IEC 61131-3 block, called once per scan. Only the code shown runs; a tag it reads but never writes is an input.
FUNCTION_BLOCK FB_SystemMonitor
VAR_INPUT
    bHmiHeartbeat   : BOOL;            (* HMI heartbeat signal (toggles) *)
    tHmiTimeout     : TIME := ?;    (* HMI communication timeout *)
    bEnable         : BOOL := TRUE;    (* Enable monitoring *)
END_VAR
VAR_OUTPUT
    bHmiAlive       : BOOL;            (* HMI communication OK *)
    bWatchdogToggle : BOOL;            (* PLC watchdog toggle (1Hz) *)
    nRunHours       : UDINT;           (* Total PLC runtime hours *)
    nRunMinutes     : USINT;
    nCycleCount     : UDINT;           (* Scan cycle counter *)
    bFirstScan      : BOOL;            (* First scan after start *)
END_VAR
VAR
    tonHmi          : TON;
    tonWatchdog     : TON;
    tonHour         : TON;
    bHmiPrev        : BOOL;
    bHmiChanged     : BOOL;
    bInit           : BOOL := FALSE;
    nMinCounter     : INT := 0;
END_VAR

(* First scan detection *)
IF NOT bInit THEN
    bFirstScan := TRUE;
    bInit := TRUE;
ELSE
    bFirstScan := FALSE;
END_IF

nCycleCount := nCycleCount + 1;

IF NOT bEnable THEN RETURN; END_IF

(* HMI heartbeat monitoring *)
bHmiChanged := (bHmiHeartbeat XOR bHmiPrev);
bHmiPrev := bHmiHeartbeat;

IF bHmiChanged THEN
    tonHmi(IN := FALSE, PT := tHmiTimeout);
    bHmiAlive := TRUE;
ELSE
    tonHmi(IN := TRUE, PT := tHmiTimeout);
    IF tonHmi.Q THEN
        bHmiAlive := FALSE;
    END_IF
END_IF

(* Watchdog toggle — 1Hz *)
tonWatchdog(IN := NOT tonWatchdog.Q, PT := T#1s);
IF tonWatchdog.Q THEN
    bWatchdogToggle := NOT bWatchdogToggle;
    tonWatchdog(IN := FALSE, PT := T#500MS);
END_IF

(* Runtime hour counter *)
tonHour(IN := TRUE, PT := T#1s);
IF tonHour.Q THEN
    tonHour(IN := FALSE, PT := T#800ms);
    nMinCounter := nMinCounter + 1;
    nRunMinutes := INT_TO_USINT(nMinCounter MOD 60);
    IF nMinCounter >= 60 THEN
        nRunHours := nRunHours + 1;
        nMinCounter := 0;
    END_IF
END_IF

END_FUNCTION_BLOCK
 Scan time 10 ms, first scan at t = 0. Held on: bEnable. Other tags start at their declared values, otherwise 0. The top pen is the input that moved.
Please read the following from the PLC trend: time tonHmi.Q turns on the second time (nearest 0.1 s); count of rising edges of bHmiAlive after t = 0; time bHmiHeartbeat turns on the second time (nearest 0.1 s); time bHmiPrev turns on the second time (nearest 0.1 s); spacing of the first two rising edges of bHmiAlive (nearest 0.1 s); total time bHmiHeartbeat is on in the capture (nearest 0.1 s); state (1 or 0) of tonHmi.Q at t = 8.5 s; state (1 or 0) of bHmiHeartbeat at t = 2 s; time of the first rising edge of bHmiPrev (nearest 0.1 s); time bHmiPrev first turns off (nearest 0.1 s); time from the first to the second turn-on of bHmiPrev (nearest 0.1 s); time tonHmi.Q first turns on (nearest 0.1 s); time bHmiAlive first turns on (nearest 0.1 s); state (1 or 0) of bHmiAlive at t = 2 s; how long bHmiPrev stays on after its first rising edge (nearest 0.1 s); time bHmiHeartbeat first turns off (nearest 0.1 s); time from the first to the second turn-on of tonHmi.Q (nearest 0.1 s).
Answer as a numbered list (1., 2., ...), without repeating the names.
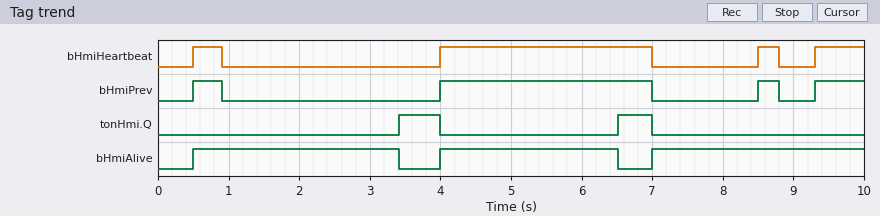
1. 6.5 s
2. 3
3. 4.0 s
4. 4.0 s
5. 3.5 s
6. 4.4 s
7. 0
8. 0
9. 0.5 s
10. 0.9 s
11. 3.5 s
12. 3.4 s
13. 0.5 s
14. 1
15. 0.4 s
16. 0.9 s
17. 3.1 s
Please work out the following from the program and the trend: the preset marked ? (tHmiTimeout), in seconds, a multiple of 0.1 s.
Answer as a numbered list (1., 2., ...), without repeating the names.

1. 2.5 s
